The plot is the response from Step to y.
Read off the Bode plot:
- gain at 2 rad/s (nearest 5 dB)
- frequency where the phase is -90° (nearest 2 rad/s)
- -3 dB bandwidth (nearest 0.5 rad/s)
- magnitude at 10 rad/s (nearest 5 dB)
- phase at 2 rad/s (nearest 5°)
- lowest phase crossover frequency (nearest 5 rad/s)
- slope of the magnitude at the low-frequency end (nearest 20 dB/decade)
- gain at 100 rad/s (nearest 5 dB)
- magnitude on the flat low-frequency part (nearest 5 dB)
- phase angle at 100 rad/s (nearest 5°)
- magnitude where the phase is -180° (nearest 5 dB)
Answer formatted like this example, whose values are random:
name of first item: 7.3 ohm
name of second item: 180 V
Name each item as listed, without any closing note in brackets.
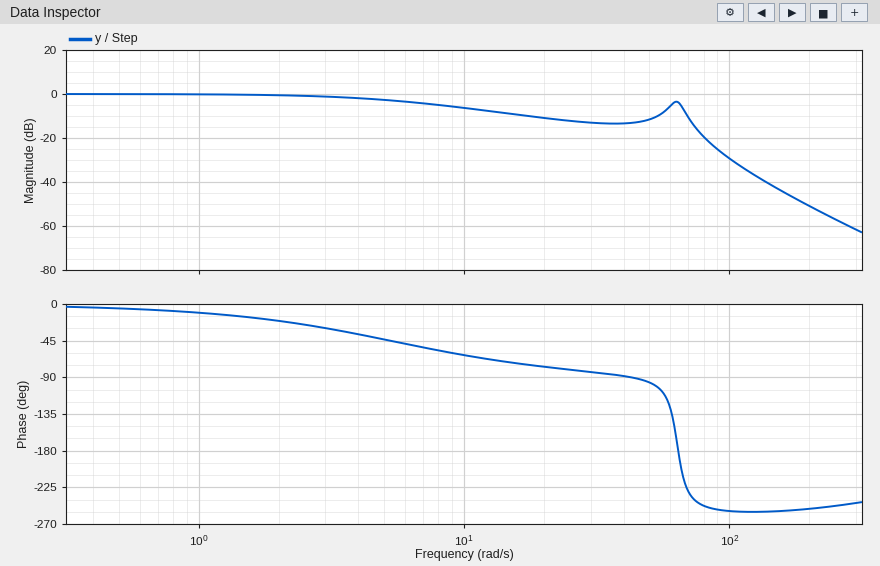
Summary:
gain at 2 rad/s: 0 dB
frequency where the phase is -90°: 42 rad/s
-3 dB bandwidth: 5.5 rad/s
magnitude at 10 rad/s: -5 dB
phase at 2 rad/s: -20°
lowest phase crossover frequency: 65 rad/s
slope of the magnitude at the low-frequency end: 0 dB/decade
gain at 100 rad/s: -30 dB
magnitude on the flat low-frequency part: 0 dB
phase angle at 100 rad/s: -255°
magnitude where the phase is -180°: -5 dB
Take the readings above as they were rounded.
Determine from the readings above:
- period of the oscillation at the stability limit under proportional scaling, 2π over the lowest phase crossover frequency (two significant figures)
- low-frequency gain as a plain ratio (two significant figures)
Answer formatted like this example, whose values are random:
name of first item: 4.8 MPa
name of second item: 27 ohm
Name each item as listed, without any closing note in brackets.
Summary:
period of the oscillation at the stability limit under proportional scaling, 2π over the lowest phase crossover frequency: 0.097 s
low-frequency gain as a plain ratio: 1.0
